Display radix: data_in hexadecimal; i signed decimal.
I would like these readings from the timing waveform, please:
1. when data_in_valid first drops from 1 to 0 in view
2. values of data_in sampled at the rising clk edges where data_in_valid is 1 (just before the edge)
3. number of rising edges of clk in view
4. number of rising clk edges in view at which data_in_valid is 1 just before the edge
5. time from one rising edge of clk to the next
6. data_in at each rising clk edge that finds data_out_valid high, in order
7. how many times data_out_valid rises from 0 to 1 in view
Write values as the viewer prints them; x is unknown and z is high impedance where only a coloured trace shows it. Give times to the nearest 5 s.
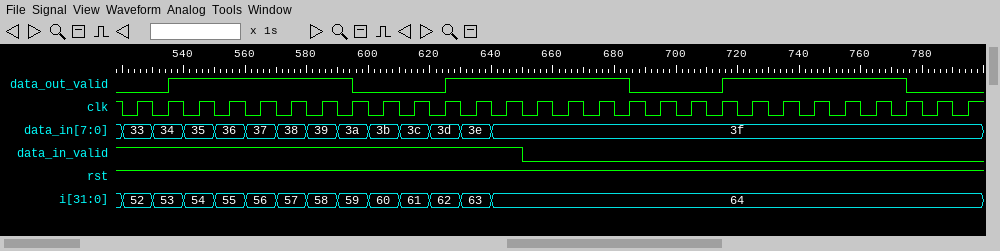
650 s
33, 34, 35, 36, 37, 38, 39, 3a, 3b, 3c, 3d, 3e, 3f
28
13
10 s
35, 36, 37, 38, 39, 3a, 3e, 3f, 3f, 3f, 3f, 3f, 3f, 3f, 3f, 3f, 3f, 3f
3
